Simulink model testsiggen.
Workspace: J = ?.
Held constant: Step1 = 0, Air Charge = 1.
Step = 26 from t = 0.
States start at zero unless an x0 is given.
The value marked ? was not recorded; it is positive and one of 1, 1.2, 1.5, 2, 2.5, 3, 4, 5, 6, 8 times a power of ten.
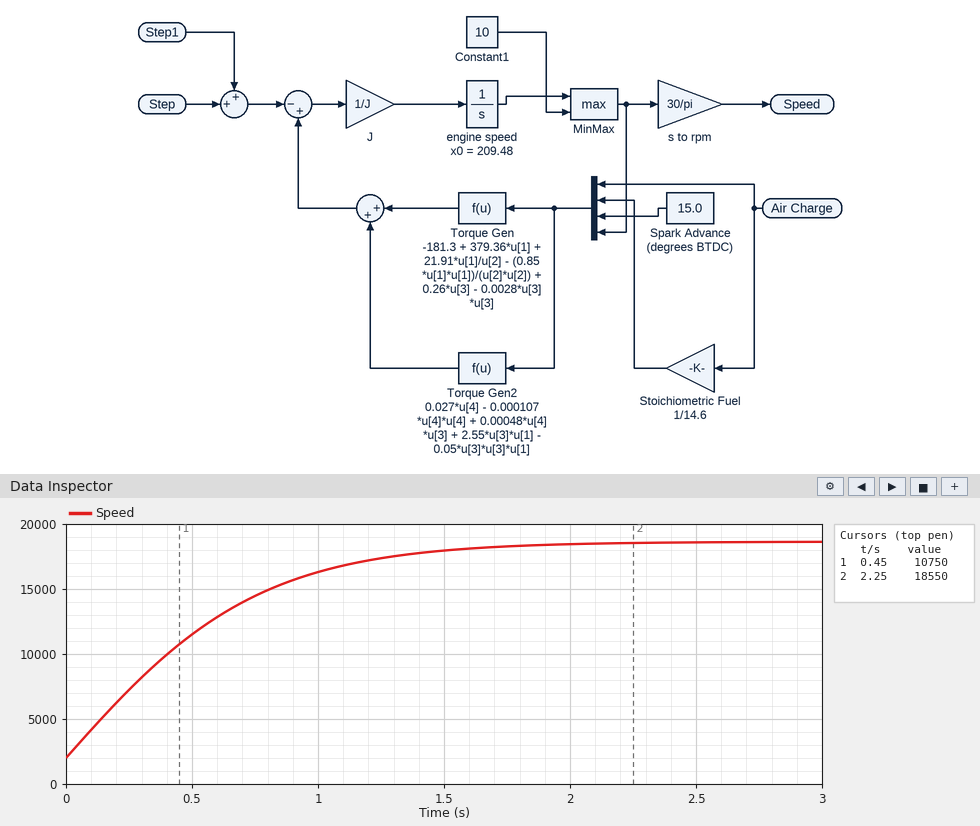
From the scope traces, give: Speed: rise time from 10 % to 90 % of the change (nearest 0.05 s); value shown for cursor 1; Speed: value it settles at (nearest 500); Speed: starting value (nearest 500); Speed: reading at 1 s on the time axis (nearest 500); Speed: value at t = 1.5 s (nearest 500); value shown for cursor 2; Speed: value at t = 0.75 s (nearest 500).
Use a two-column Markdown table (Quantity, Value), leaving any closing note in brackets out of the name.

| Quantity | Value |
|---|---|
| Speed: rise time from 10 % to 90 % of the change | 1.05 s |
| value shown for cursor 1 | 10750 |
| Speed: value it settles at | 18500 |
| Speed: starting value | 2000 |
| Speed: reading at 1 s on the time axis | 16500 |
| Speed: value at t = 1.5 s | 18000 |
| value shown for cursor 2 | 18550 |
| Speed: value at t = 0.75 s | 14500 |
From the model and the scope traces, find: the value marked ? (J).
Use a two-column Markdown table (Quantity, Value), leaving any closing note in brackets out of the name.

| Quantity | Value |
|---|---|
| the value marked ? | 0.15 |
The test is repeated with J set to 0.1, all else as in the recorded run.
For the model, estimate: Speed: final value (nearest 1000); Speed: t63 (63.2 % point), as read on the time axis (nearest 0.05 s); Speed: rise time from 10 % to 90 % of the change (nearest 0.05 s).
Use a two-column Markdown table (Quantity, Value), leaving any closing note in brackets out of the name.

| Quantity | Value |
|---|---|
| Speed: final value | 19000 |
| Speed: t63 (63.2 % point), as read on the time axis | 0.40 s |
| Speed: rise time from 10 % to 90 % of the change | 0.70 s |
